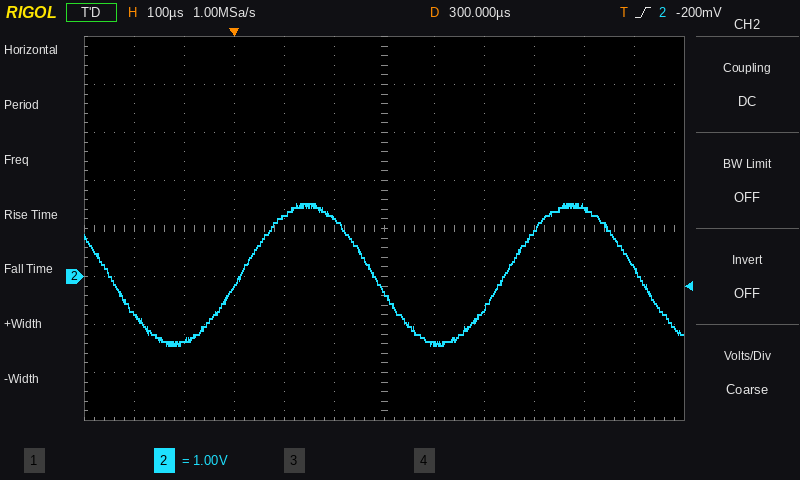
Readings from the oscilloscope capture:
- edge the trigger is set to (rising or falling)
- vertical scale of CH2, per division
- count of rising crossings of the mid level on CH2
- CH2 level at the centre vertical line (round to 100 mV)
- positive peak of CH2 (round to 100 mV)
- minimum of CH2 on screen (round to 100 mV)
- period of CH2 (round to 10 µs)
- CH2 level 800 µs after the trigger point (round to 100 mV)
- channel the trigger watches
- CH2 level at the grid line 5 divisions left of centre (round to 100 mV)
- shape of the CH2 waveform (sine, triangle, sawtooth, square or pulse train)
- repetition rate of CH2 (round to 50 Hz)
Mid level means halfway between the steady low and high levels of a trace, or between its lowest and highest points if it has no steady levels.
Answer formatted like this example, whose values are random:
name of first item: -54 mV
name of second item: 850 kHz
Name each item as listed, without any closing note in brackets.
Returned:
edge the trigger is set to: rising
vertical scale of CH2, per division: 1 V
count of rising crossings of the mid level on CH2: 2
CH2 level at the centre vertical line: -300 mV
positive peak of CH2: 1.5 V
minimum of CH2 on screen: -1.4 V
period of CH2: 530 µs
CH2 level 800 µs after the trigger point: 200 mV
channel the trigger watches: CH2
CH2 level at the grid line 5 divisions left of centre: -800 mV
shape of the CH2 waveform: sine
repetition rate of CH2: 1.90 kHz
